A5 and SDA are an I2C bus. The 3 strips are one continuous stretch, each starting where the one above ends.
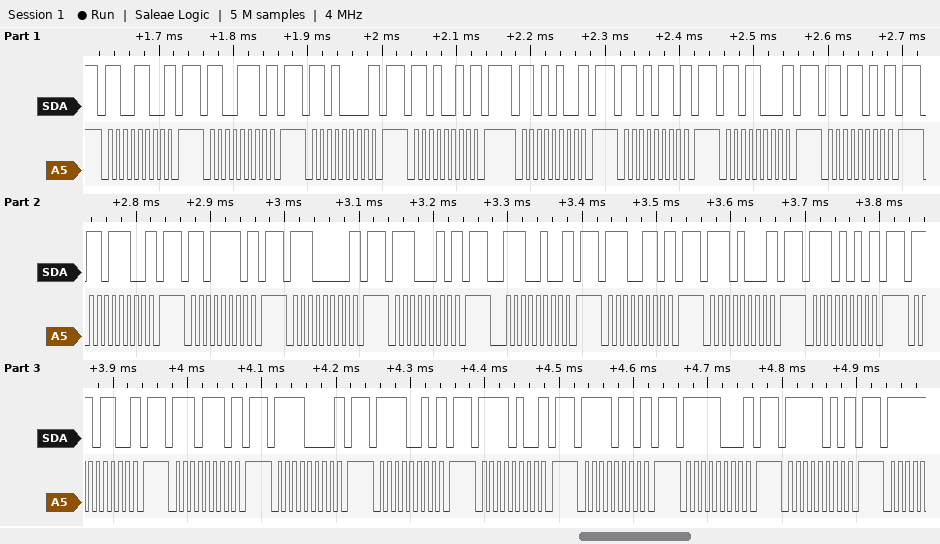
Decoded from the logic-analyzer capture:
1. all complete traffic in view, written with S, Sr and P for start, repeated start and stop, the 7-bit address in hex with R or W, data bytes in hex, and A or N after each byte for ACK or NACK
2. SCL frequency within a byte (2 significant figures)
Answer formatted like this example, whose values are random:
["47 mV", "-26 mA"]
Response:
["S 66W N P S 67W N P S 68W N P S 69W N P S 6AW N P S 6BW N P S 6CW N P S 6DW N P S 6EW N P S 6FW N P S 70W N P S 71W N P S 72W N P S 73W N P S 74W N P S 75W N P S 76W N P S 77W N P S 78W N P S 79W N P S 7AW N P S 7BW N P S 7CW N P S 7DW N P", "100 kHz"]
